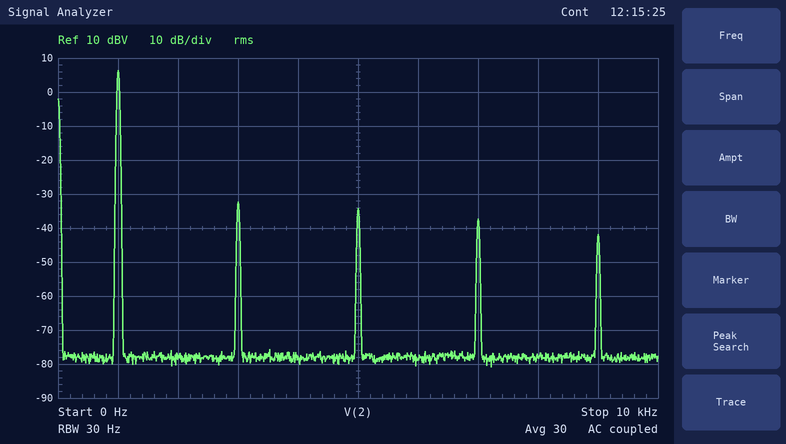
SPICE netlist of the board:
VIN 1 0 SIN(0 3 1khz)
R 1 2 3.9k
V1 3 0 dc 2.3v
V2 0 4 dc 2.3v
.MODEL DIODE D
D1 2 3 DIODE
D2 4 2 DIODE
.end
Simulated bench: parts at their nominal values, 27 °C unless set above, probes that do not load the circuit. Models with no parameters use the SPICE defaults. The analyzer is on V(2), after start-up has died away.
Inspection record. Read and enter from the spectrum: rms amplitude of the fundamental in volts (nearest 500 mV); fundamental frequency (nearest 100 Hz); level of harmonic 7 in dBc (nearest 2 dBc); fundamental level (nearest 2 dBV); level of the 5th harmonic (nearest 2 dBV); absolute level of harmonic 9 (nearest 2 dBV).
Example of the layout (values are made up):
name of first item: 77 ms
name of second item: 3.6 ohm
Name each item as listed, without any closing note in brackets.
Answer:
rms amplitude of the fundamental in volts: 2.0 V
fundamental frequency: 1.0 kHz
level of harmonic 7 in dBc: -44 dBc
fundamental level: 6 dBV
level of the 5th harmonic: -34 dBV
absolute level of harmonic 9: -42 dBV
